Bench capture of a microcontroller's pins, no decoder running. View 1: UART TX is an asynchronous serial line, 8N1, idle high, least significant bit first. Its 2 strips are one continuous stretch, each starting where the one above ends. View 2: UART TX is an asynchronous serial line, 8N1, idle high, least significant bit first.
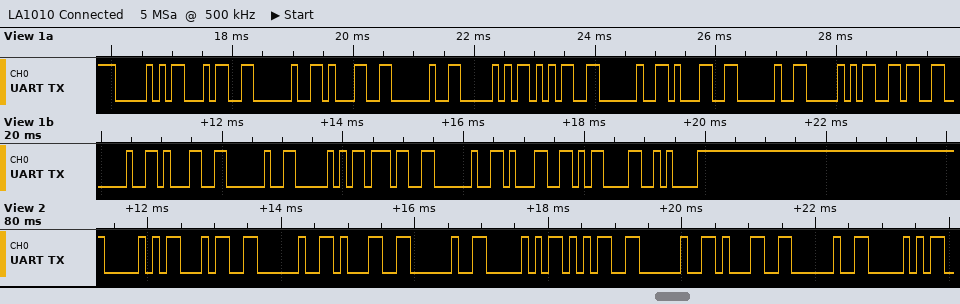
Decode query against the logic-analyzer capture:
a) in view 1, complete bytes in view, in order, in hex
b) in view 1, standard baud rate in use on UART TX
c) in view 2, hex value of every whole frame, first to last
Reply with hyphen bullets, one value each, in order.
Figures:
- 50 34 20 31 20 50 35 20 31 20 50 36 20 31 20 50 37 20 31 0D 0A
- 9600 baud
- 50 34 20 31 20 50 35 20 31 20 50
